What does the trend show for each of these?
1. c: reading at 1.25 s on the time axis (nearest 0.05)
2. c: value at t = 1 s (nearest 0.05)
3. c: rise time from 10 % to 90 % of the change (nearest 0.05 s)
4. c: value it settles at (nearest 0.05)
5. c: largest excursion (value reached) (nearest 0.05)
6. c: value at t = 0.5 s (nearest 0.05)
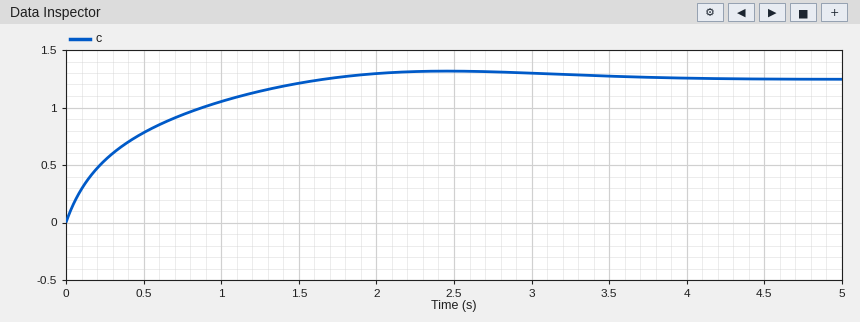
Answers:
1.15
1.05
1.15 s
1.25
1.30
0.80
